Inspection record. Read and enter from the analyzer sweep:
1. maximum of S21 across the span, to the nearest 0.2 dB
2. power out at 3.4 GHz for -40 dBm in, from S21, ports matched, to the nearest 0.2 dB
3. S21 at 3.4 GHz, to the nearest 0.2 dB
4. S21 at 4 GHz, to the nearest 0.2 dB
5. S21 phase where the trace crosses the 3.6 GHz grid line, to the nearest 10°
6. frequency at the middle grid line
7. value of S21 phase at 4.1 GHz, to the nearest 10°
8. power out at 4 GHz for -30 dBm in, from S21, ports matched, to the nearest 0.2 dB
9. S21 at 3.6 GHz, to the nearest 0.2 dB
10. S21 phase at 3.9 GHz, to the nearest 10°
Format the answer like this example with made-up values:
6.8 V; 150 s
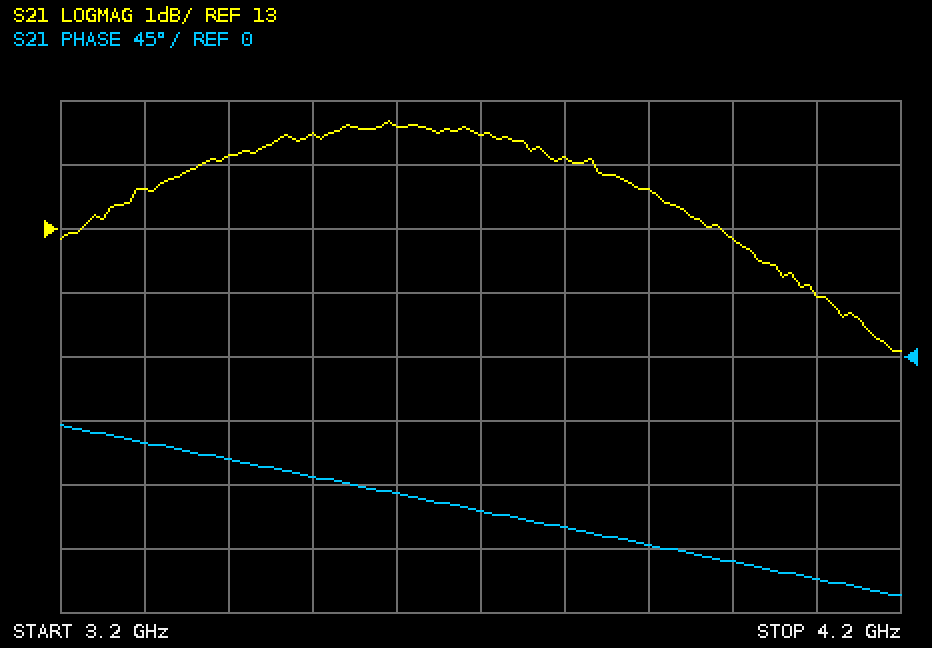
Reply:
14.6 dB; -25.8 dBm; 14.2 dB; 12.8 dB; -100°; 3.7 GHz; -160°; -17.2 dBm; 14.6 dB; -130°
